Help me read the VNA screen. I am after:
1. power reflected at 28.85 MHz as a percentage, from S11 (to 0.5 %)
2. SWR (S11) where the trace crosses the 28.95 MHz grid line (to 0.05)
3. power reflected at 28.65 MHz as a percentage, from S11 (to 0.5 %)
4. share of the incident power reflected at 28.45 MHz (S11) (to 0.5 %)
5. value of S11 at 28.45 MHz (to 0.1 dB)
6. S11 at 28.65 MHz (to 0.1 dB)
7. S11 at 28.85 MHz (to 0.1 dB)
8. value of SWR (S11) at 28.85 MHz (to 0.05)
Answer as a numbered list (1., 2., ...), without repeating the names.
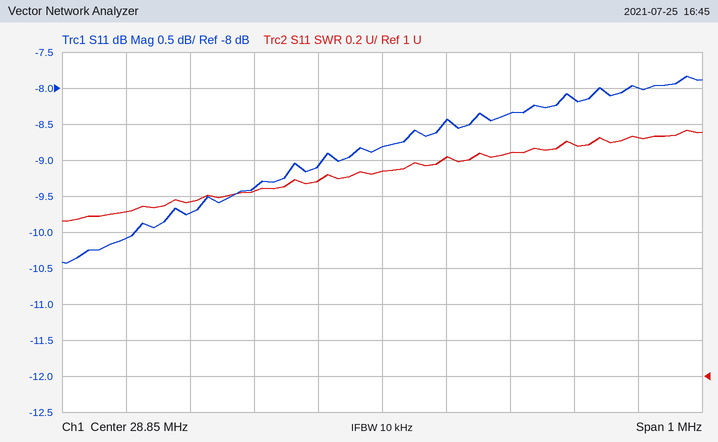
1. 13.0 %
2. 2.20
3. 11.5 %
4. 10.0 %
5. -10.1 dB
6. -9.4 dB
7. -8.8 dB
8. 2.15
